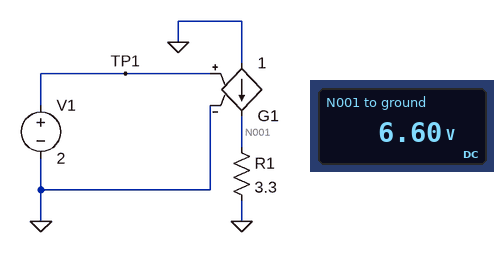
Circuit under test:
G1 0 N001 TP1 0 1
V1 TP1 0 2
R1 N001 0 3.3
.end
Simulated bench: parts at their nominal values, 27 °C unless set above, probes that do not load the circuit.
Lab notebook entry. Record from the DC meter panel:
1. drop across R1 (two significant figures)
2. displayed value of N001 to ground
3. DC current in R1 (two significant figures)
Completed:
6.6 V
6.60 V
2.0 A
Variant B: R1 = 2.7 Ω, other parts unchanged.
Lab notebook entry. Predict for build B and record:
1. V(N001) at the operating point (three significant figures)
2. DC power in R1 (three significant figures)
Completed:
5.40 V
10.8 W
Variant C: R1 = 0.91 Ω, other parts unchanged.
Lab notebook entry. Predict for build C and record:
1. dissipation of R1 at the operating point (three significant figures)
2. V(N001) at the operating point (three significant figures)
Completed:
3.64 W
1.82 V
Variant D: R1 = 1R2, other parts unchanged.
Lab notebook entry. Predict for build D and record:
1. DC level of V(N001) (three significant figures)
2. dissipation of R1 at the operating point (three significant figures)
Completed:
2.40 V
4.80 W
